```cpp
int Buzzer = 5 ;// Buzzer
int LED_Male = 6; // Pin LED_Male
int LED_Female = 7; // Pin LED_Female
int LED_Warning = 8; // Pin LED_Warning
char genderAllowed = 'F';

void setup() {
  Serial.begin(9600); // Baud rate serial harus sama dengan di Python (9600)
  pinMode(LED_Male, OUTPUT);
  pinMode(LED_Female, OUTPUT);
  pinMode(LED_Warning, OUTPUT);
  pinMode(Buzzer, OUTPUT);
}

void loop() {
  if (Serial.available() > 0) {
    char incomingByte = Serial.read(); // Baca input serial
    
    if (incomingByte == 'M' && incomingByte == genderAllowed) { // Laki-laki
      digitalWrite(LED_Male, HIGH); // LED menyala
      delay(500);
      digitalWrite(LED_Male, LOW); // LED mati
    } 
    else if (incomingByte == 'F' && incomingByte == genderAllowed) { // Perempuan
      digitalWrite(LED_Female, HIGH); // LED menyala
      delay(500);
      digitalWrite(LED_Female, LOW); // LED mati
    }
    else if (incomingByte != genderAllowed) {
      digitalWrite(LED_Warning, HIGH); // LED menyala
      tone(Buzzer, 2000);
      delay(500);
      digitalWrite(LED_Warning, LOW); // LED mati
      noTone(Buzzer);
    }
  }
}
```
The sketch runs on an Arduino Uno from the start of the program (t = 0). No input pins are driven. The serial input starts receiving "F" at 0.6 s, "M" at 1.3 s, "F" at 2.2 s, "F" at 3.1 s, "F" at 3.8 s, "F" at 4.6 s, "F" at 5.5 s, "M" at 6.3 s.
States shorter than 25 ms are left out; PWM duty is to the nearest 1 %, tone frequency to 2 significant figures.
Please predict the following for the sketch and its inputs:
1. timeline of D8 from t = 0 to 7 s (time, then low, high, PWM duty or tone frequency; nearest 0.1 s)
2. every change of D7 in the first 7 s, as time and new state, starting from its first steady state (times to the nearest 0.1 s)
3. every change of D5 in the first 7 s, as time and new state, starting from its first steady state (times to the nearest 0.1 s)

0 s low; 1.3 s high; 1.8 s low; 6.3 s high; 6.8 s low
0 s low; 0.6 s high; 1.1 s low; 2.2 s high; 2.7 s low; 3.1 s high; 3.6 s low; 3.8 s high; 4.3 s low; 4.6 s high; 5.1 s low; 5.5 s high; 6 s low
0 s low; 1.3 s tone 2000 Hz; 1.8 s low; 6.3 s tone 2000 Hz; 6.8 s low
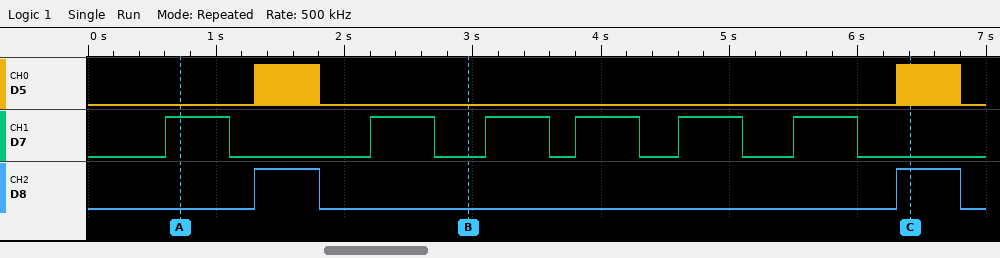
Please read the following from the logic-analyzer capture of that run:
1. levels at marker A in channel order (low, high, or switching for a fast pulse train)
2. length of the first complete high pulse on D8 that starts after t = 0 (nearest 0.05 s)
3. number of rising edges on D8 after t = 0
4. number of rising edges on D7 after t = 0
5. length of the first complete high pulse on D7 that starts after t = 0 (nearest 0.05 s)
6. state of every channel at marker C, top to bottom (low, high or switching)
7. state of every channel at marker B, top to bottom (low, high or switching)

D5 low, D7 high, D8 low
0.50 s
2
6
0.50 s
D5 switching, D7 low, D8 high
D5 low, D7 low, D8 low
